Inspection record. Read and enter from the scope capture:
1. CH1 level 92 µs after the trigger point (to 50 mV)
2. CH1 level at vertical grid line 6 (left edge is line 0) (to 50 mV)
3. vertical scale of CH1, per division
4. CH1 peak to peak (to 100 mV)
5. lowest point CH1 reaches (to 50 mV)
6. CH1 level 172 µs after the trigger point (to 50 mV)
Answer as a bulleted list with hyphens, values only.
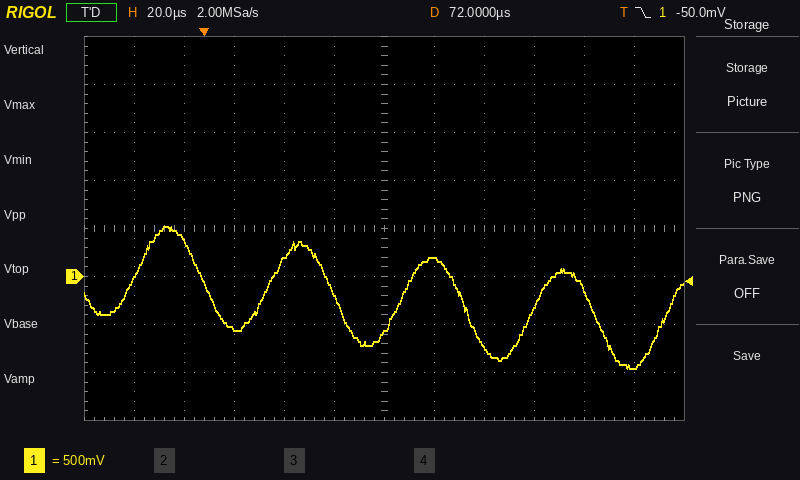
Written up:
- 200 mV
- -600 mV
- 500 mV
- 1.50 V
- -950 mV
- -950 mV
